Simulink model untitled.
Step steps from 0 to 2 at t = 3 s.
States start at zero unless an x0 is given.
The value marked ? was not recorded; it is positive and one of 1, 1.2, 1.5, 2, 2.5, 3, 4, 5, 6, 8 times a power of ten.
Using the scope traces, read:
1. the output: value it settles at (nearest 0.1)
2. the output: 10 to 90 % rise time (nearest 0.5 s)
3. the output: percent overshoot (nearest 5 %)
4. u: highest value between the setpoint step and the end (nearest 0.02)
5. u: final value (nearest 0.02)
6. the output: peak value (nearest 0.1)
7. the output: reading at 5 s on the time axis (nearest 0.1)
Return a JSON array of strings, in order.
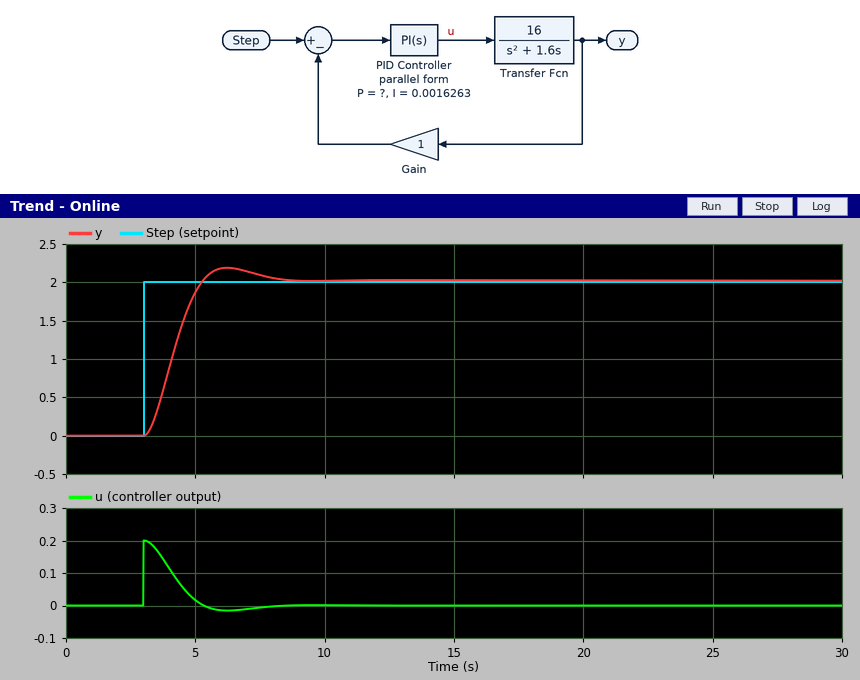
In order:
["2.0", "1.5 s", "10 %", "0.20", "0.00", "2.2", "1.9"]
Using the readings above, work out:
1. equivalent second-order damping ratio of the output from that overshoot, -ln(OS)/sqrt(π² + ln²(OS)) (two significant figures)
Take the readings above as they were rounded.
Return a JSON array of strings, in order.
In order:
["0.59"]
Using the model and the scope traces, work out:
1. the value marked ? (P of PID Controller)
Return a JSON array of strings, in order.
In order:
["0.1"]
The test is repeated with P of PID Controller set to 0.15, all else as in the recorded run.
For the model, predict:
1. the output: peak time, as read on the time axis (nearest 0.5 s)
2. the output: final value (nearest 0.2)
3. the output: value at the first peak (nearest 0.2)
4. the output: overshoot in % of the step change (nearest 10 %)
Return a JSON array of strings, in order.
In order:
["5.5 s", "2.0", "2.4", "20 %"]
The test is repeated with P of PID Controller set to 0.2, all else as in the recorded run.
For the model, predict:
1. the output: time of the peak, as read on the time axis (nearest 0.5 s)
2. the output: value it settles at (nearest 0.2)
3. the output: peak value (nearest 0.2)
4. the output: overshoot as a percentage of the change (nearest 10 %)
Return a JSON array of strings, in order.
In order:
["5.0 s", "2.0", "2.4", "20 %"]
